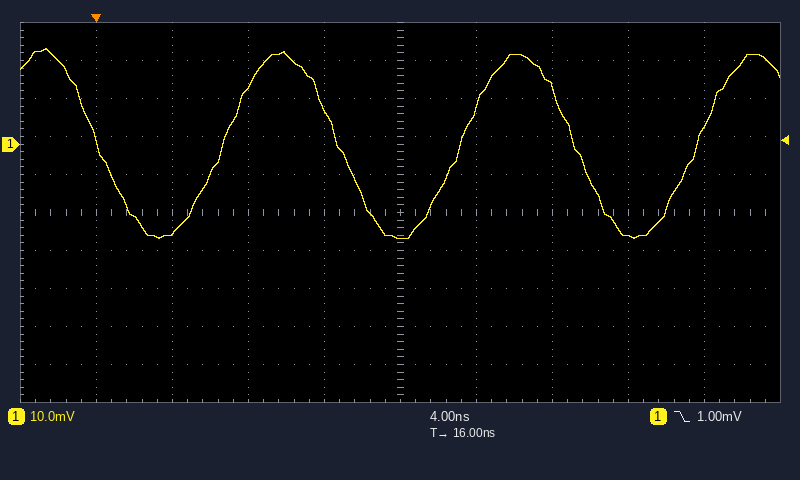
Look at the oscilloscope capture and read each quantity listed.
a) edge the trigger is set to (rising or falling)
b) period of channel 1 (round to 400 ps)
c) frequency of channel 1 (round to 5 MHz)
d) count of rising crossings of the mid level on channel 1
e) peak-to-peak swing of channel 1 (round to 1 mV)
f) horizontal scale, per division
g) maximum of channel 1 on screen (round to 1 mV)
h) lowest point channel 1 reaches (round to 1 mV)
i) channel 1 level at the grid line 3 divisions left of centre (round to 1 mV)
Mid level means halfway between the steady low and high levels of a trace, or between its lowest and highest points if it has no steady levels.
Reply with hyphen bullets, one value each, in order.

- falling
- 12.4 ns
- 80 MHz
- 3
- 50 mV
- 4 ns
- 25 mV
- -25 mV
- -23 mV
